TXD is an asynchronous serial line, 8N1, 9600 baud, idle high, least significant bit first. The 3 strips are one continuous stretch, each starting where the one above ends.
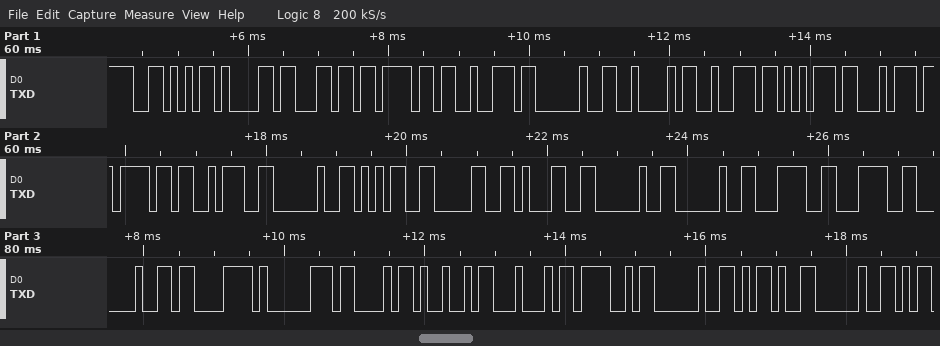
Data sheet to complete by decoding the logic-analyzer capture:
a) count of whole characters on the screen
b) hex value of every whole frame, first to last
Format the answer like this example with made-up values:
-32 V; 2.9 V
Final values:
30; 56 61 6C 6F 72 20 42 72 75 74 6F 3A 20 35 30 31 20 20 3C 3C 20 C3 81 43 49 44 4F 20 2D 20
